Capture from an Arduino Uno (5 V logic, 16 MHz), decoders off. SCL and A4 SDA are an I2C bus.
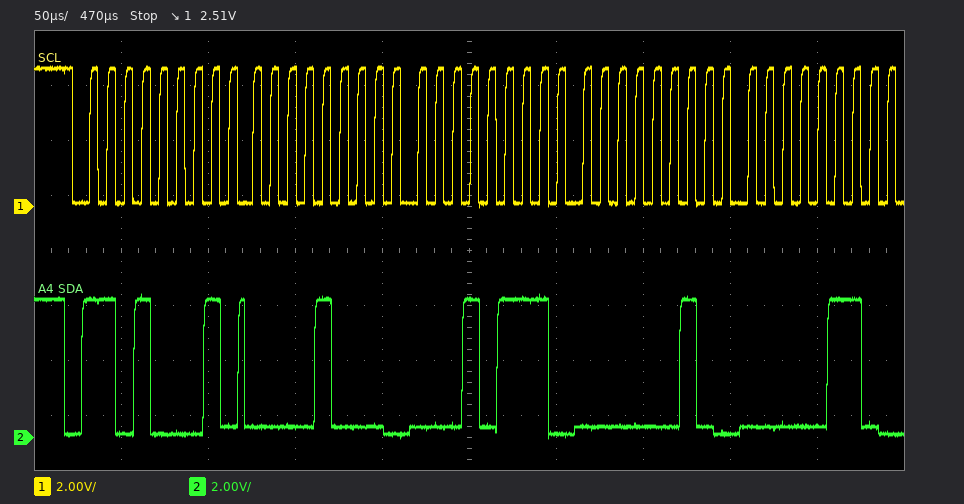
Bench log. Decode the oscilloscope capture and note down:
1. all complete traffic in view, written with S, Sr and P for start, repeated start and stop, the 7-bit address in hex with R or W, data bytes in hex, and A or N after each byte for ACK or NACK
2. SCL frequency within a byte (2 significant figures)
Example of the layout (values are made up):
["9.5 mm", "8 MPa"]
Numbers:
["S 68R A 08 A 17 A 02 A 06 A", "100 kHz"]
